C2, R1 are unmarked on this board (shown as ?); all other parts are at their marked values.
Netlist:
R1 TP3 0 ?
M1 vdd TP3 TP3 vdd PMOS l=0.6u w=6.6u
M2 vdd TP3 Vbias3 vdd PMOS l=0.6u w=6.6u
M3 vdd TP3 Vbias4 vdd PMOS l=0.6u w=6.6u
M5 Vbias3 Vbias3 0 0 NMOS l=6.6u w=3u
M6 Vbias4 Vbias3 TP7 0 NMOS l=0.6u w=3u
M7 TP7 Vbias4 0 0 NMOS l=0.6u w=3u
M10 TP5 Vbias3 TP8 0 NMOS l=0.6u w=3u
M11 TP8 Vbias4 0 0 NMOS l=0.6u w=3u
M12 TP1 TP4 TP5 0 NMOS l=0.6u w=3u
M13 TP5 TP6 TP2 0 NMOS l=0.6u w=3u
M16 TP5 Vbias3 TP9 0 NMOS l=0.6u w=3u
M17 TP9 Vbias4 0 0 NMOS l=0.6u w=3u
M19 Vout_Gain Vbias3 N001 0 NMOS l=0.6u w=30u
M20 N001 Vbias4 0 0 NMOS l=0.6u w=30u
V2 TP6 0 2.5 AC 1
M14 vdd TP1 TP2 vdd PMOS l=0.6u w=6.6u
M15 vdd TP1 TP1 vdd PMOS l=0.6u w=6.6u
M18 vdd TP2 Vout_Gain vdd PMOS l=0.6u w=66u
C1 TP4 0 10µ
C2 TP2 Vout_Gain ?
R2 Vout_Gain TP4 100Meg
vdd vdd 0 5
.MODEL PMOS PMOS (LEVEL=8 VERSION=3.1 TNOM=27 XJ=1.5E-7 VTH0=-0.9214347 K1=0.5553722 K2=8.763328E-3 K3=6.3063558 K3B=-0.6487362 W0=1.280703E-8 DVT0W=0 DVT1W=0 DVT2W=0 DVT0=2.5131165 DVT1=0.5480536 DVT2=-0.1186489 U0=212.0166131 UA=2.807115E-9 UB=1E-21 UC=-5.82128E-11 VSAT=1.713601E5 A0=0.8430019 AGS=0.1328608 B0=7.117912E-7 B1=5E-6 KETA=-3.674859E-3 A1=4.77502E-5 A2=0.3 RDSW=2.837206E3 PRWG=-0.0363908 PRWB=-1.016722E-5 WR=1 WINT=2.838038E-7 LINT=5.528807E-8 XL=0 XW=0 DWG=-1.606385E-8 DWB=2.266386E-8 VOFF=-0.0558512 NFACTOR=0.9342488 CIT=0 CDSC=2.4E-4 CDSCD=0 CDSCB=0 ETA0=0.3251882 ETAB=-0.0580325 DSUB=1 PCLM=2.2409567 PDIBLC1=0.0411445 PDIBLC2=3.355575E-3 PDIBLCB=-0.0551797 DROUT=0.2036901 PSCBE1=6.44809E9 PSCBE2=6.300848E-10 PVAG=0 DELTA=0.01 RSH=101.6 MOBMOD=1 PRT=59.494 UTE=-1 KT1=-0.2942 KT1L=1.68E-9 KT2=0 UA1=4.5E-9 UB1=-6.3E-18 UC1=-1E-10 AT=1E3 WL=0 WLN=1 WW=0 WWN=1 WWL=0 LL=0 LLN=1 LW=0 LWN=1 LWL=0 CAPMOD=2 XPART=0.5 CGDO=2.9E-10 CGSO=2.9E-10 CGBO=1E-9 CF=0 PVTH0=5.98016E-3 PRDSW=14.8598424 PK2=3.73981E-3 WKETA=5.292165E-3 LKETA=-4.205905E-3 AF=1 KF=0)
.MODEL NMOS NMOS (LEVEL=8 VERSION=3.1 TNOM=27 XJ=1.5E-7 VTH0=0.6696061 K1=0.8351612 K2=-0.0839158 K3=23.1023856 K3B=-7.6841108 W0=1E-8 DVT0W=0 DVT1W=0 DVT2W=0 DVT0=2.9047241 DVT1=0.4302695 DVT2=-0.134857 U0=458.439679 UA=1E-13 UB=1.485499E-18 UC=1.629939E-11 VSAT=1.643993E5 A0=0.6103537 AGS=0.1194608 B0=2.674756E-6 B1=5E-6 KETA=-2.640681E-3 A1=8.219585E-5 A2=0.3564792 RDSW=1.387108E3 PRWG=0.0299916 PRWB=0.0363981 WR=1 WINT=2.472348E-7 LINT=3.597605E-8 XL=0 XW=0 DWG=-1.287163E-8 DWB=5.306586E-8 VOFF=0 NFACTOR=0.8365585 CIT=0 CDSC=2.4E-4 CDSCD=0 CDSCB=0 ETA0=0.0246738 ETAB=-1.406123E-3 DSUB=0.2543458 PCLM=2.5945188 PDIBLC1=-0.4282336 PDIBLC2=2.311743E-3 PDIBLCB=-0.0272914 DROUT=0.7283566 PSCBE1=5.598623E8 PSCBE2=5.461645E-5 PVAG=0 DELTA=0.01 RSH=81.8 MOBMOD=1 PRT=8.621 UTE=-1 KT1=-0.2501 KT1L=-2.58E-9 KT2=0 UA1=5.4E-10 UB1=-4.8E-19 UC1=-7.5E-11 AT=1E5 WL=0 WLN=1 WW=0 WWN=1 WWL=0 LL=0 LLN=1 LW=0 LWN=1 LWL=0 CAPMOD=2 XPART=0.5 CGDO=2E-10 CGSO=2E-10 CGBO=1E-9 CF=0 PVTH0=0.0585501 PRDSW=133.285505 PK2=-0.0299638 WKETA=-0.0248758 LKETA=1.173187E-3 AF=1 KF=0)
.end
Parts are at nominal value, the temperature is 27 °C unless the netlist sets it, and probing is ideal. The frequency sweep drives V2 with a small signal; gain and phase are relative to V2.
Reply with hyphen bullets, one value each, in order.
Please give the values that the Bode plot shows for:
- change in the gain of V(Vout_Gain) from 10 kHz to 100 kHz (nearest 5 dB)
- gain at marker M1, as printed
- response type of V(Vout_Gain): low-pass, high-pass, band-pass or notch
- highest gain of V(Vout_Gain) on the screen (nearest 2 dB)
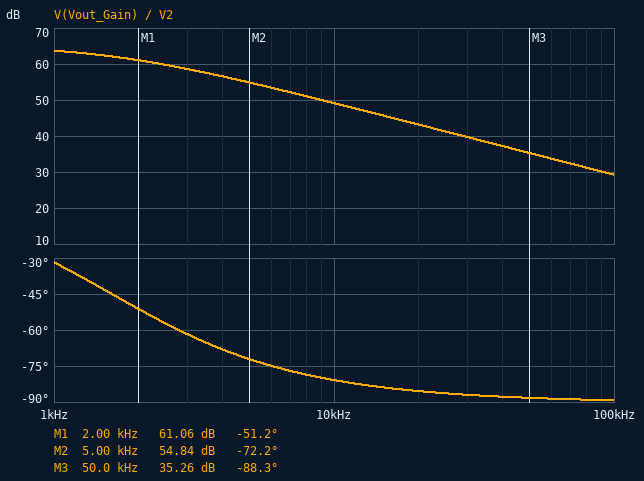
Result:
- -20 dB
- 61.06 dB
- low-pass
- 64 dB
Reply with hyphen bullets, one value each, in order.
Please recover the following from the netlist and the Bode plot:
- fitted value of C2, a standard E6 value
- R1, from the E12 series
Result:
- 22 pF
- 100 kΩ
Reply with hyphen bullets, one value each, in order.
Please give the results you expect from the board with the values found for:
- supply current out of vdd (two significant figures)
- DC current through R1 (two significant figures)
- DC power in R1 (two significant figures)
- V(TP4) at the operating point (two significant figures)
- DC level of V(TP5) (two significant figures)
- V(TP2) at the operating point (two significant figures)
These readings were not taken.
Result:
- 1.1 mA
- 37 µA
- 140 µW
- 2.5 V
- 1.1 V
- 3.6 V
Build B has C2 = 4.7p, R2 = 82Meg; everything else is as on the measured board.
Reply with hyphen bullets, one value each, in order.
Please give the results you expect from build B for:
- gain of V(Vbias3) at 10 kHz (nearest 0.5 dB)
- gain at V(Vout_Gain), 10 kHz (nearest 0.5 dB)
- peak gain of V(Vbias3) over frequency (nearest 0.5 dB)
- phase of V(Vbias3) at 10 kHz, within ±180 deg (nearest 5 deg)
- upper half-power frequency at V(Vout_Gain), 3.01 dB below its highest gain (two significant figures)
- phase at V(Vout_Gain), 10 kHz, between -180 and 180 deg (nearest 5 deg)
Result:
- -42.5 dB
- 60.5 dB
- -40.5 dB
- 35 deg
- 7.5 kHz
- -55 deg
